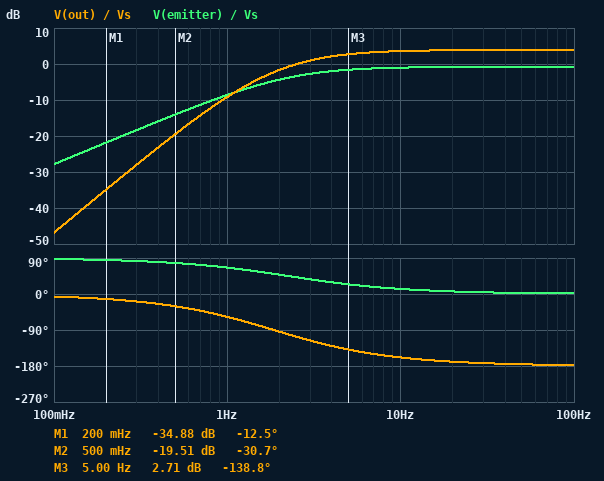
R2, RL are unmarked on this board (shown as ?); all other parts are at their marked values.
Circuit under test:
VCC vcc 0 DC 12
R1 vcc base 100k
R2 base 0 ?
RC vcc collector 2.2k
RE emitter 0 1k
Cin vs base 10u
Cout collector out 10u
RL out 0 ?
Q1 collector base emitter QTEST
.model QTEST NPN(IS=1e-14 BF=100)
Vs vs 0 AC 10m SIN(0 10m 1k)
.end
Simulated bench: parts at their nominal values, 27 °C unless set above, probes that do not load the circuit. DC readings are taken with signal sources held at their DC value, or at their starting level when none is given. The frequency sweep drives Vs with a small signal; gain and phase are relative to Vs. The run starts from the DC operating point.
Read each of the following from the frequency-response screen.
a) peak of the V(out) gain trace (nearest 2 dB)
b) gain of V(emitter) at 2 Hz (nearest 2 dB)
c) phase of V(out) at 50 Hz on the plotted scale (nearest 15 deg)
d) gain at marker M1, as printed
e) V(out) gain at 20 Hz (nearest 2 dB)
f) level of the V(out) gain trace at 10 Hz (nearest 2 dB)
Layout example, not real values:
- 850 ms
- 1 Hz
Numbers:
- 4 dB
- -4 dB
- -180 deg
- -34.88 dB
- 4 dB
- 4 dB
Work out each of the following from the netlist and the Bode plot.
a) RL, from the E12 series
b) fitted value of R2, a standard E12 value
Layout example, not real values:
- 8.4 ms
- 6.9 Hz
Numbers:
- 8.2 kΩ
- 8.2 kΩ
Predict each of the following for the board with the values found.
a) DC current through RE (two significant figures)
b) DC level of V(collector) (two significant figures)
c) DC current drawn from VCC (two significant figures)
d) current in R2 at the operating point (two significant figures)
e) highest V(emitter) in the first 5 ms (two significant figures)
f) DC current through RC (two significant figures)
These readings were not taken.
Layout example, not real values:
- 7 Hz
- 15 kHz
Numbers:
- 270 µA
- 11 V
- 380 µA
- 110 µA
- 280 mV
- 270 µA
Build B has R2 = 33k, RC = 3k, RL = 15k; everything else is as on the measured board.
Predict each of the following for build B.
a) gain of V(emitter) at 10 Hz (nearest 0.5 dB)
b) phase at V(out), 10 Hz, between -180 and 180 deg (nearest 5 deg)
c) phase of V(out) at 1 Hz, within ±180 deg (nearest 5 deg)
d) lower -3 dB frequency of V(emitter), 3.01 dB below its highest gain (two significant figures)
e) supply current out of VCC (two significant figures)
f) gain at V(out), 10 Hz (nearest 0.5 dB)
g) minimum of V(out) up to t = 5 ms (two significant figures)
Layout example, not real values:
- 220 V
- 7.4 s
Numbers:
- 0 dB
- -170 deg
- -100 deg
- 800 mHz
- 1.9 mA
- 7.5 dB
- -24 mV
